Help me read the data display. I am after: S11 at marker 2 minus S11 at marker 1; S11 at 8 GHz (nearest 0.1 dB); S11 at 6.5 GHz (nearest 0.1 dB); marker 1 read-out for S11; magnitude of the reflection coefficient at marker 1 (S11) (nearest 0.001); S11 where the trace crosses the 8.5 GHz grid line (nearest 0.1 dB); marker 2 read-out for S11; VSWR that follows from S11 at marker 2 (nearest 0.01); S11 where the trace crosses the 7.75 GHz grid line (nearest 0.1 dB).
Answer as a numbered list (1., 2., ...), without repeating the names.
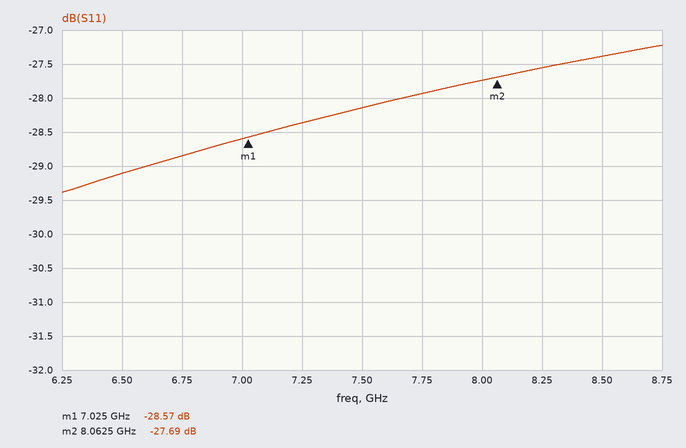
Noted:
1. 0.88 dB
2. -27.7 dB
3. -29.1 dB
4. -28.57 dB
5. 0.037
6. -27.4 dB
7. -27.69 dB
8. 1.09
9. -27.9 dB
